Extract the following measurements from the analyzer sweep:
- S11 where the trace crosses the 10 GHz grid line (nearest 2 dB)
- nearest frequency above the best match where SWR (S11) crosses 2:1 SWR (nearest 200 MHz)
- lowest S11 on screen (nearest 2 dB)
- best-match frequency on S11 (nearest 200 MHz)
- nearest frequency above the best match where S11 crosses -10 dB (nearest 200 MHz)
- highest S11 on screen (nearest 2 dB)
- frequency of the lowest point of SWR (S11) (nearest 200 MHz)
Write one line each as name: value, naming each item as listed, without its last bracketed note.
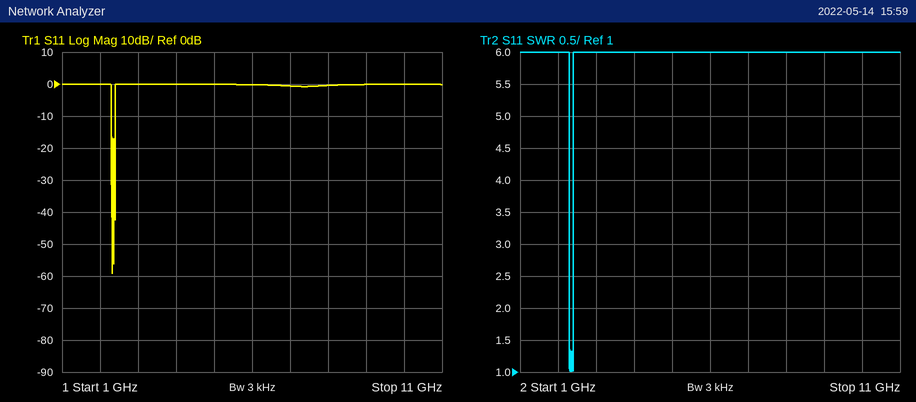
S11 where the trace crosses the 10 GHz grid line: 0 dB
nearest frequency above the best match where SWR (S11) crosses 2:1 SWR: 2.4 GHz
lowest S11 on screen: -60 dB
best-match frequency on S11: 2.4 GHz
nearest frequency above the best match where S11 crosses -10 dB: 2.4 GHz
highest S11 on screen: 0 dB
frequency of the lowest point of SWR (S11): 2.4 GHz
